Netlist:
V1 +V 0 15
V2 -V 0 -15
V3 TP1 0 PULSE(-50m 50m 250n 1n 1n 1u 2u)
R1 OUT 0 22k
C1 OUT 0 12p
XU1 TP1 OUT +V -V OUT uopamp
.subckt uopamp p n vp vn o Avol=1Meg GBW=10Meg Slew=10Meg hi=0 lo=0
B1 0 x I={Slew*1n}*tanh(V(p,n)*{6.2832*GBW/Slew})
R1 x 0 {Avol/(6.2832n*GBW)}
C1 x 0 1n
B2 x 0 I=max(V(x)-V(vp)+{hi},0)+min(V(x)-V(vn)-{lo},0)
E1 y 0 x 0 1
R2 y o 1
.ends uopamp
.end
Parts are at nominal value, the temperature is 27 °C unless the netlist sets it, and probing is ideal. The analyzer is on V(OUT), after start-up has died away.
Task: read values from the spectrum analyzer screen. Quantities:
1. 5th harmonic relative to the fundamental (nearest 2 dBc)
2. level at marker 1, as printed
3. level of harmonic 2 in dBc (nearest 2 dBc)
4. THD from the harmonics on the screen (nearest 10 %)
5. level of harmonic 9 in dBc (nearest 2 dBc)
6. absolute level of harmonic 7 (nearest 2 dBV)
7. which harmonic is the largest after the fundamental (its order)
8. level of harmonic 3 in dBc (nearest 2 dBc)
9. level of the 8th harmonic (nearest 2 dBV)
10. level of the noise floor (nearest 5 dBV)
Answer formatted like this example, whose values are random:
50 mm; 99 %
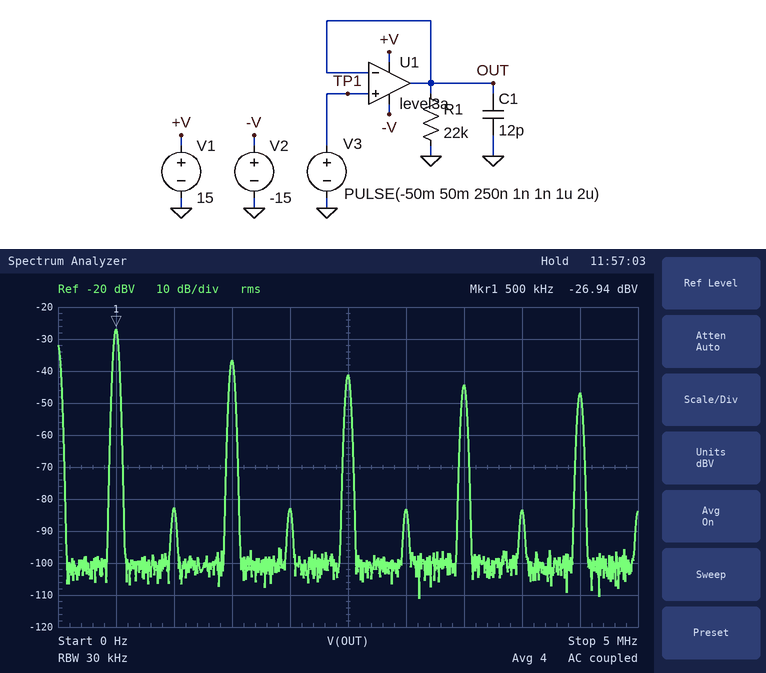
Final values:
-14 dBc; -26.94 dBV; -56 dBc; 40 %; -20 dBc; -44 dBV; 3; -10 dBc; -84 dBV; -100 dBV
